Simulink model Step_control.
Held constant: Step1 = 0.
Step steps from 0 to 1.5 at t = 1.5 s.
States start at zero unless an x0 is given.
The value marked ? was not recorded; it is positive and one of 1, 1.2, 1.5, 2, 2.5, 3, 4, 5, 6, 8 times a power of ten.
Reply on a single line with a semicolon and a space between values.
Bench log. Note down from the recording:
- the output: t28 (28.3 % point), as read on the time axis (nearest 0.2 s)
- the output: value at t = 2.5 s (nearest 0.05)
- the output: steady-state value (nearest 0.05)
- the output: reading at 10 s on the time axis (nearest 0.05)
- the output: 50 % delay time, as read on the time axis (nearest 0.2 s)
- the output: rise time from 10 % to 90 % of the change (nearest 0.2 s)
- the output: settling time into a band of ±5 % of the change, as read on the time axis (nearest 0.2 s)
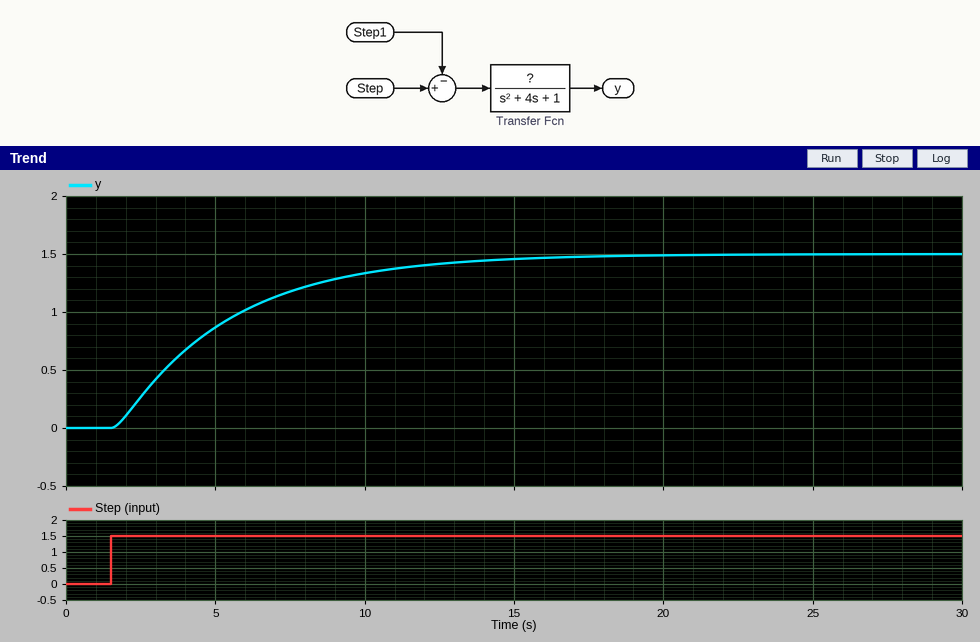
3.0 s; 0.25; 1.50; 1.35; 4.4 s; 8.2 s; 13.0 s
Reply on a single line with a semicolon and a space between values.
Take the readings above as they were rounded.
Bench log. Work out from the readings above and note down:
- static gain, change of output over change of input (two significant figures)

1.0
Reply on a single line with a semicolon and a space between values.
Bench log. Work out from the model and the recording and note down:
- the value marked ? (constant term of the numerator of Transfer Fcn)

1
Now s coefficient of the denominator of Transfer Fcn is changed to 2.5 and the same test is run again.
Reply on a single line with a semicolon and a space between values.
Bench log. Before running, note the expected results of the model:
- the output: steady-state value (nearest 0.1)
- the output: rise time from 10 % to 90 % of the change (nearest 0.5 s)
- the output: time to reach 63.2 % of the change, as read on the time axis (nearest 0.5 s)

1.5; 4.5 s; 4.0 s
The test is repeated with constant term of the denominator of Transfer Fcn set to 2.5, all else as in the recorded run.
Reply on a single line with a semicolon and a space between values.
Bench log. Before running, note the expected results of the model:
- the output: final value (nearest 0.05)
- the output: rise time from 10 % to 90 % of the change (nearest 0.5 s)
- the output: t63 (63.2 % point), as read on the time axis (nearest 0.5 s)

0.60; 3.0 s; 3.0 s
